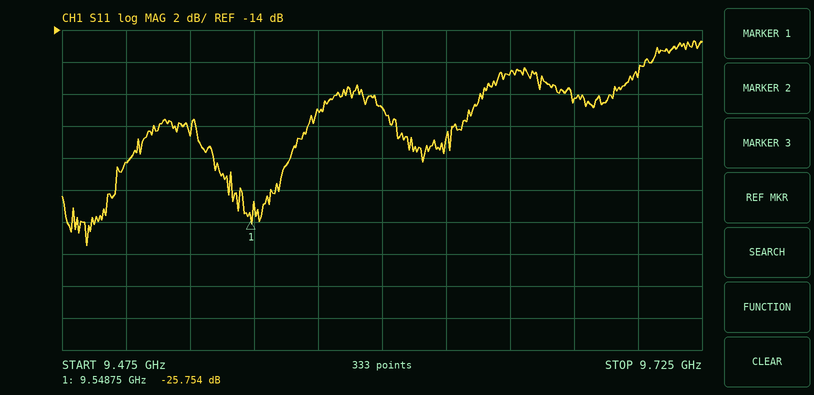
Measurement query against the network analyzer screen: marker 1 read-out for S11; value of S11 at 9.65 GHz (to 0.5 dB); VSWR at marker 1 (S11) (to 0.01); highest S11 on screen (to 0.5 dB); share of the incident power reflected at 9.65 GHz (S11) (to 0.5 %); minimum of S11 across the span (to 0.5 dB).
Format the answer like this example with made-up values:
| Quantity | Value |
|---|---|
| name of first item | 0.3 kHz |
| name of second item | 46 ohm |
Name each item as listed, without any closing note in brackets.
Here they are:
| Quantity | Value |
|---|---|
| marker 1 read-out for S11 | -25.754 dB |
| value of S11 at 9.65 GHz | -16.5 dB |
| VSWR at marker 1 (S11) | 1.11 |
| highest S11 on screen | -14.5 dB |
| share of the incident power reflected at 9.65 GHz (S11) | 2.0 % |
| minimum of S11 across the span | -27.5 dB |
